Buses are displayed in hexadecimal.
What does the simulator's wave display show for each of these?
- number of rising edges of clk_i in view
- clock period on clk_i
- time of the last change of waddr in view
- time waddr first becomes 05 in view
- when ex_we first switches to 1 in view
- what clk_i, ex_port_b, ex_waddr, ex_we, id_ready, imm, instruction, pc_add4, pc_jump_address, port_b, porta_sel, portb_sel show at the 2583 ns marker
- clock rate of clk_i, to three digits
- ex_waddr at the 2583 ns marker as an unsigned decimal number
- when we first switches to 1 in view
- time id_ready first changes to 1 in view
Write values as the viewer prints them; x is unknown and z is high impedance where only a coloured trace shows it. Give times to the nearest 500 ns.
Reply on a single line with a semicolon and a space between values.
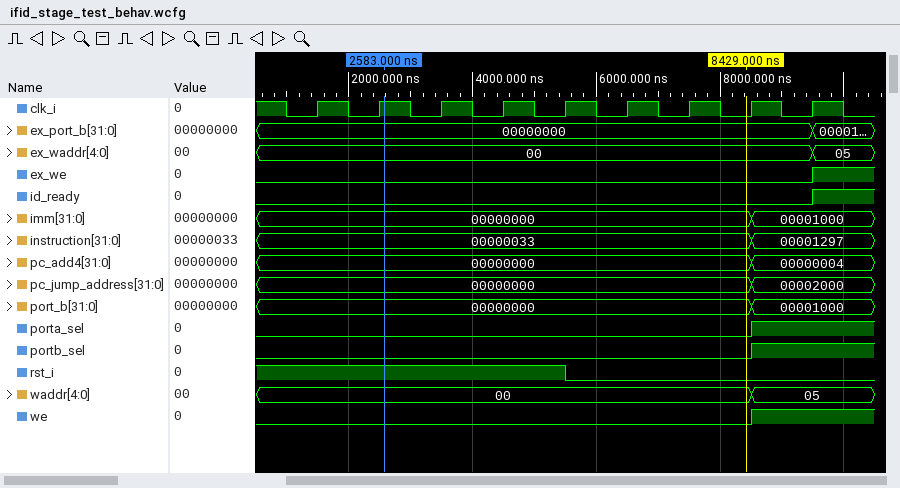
9; 1000 ns; 8500 ns; 8500 ns; 9500 ns; clk_i=1, ex_port_b=00000000, ex_waddr=00, ex_we=0, id_ready=0, imm=00000000, instruction=00000033, pc_add4=00000000, pc_jump_address=00000000, port_b=00000000, porta_sel=0, portb_sel=0; 1.00 MHz; 0; 8500 ns; 9500 ns
